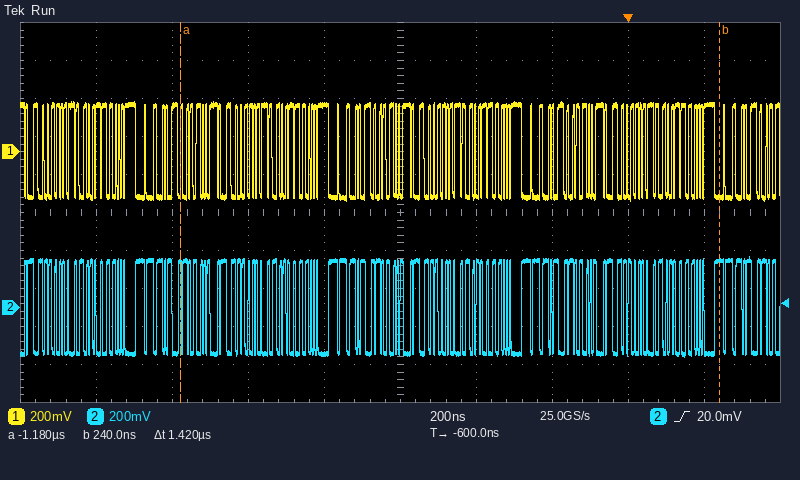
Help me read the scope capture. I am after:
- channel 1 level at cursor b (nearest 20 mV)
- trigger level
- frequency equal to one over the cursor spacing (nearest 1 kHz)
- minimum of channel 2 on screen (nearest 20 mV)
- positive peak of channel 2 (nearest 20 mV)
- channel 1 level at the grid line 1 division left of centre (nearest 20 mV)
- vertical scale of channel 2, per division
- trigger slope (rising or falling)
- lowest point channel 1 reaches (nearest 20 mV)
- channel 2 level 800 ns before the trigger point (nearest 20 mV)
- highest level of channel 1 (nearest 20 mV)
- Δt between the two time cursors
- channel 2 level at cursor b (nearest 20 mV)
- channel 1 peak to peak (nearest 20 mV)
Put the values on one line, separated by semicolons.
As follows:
-240 mV; 20.0 mV; 704 kHz; -260 mV; 260 mV; 240 mV; 200 mV; rising; -260 mV; -240 mV; 260 mV; 1.42 µs; 240 mV; 520 mV
